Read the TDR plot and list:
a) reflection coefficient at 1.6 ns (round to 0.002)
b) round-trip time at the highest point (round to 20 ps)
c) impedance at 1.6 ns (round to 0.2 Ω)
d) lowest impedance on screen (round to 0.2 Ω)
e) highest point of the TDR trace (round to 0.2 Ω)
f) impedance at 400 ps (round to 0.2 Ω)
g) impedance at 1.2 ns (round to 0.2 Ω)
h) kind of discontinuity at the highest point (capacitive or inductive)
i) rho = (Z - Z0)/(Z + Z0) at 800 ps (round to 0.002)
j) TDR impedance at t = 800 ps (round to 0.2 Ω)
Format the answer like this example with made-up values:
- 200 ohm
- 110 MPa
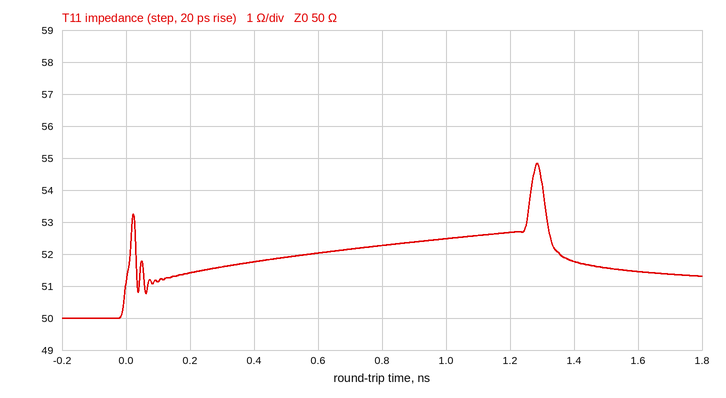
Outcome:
- +0.014
- 1.28 ns
- 51.4 Ω
- 50.0 Ω
- 54.8 Ω
- 51.8 Ω
- 52.6 Ω
- inductive
- +0.022
- 52.2 Ω
